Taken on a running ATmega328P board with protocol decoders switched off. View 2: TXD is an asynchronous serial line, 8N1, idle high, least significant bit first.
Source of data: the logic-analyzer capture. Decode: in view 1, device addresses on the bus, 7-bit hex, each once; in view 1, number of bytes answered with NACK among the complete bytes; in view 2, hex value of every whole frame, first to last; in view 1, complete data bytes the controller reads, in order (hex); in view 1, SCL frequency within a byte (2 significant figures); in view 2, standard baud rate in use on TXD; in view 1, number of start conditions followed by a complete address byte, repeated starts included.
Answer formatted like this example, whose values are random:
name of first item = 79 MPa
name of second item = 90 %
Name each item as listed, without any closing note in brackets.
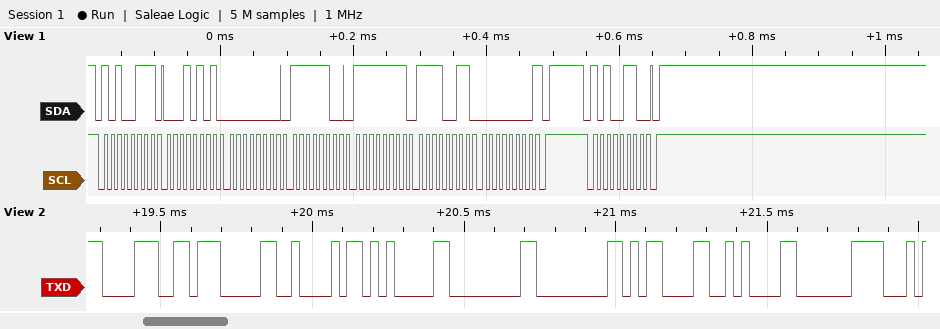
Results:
in view 1, device addresses on the bus, 7-bit hex, each once = 0x53
in view 1, number of bytes answered with NACK among the complete bytes = 1
in view 2, hex value of every whole frame, first to last = 0x38 0x07 0x42 0x05 0x00 0x00 0x0D 0x0A 0xC0
in view 1, complete data bytes the controller reads, in order = 15 00 FC FF F3 00
in view 1, SCL frequency within a byte = 100 kHz
in view 2, standard baud rate in use on TXD = 38400 baud
in view 1, number of start conditions followed by a complete address byte, repeated starts included = 2
